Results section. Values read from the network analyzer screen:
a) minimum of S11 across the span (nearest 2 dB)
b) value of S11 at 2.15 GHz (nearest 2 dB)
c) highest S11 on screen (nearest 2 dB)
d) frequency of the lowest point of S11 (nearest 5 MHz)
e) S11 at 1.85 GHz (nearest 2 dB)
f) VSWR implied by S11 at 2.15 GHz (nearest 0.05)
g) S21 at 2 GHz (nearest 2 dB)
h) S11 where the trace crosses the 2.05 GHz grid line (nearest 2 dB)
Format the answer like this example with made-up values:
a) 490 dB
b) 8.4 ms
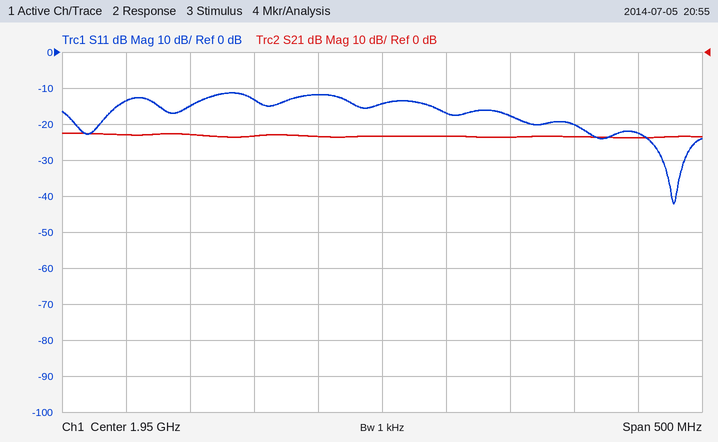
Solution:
a) -42 dB
b) -22 dB
c) -12 dB
d) 2.180 GHz
e) -14 dB
f) 1.15
g) -24 dB
h) -18 dB
